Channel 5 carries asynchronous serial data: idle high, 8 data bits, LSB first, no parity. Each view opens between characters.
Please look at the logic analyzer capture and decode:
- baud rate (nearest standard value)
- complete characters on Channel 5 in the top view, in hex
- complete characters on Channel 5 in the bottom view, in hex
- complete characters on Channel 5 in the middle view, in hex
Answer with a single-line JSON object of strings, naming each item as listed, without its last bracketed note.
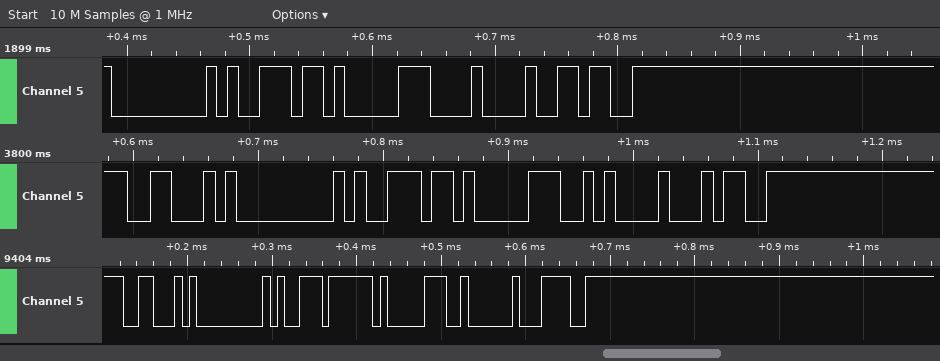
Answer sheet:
{"baud rate": "115200 baud", "complete characters on Channel 5 in the top view, in hex": "00, B9, C1, 08, 36", "complete characters on Channel 5 in the bottom view, in hex": "46, 00, B9, C1, 02, 3C", "complete characters on Channel 5 in the middle view, in hex": "46, 00, B9, C1, 0A, 34"}
